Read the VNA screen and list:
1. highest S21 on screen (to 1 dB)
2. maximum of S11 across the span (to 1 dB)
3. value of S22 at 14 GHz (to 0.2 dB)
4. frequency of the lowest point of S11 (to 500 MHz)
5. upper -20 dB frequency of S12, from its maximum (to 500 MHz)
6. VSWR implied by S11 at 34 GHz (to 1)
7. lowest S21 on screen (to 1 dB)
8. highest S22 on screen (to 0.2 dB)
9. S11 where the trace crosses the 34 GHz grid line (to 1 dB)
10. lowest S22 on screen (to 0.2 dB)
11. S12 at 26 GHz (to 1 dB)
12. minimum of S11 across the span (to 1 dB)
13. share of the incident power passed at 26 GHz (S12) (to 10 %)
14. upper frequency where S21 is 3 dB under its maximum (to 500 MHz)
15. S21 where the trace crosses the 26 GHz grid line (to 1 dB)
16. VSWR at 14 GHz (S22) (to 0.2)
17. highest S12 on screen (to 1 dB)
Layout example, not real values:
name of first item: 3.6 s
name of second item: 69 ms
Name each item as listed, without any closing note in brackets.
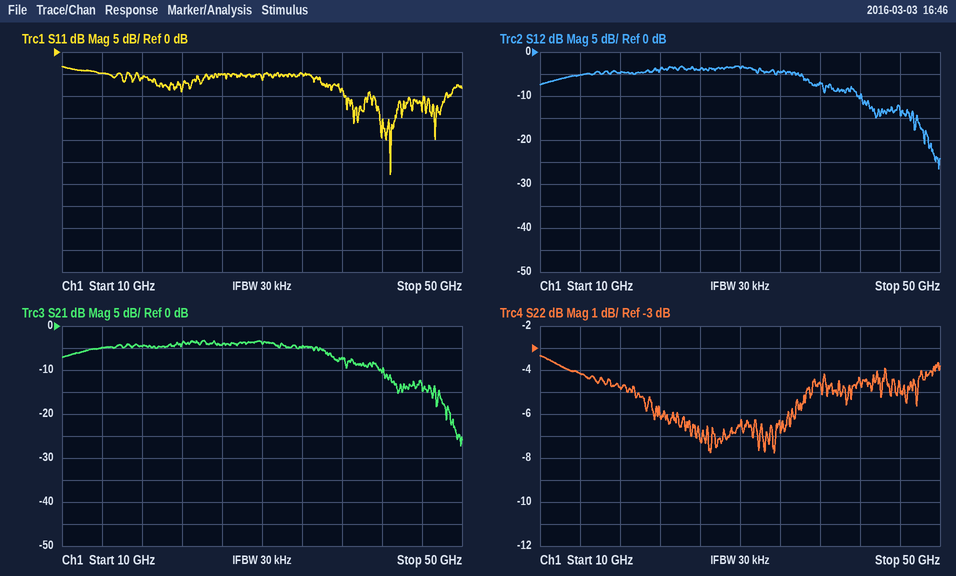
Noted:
highest S21 on screen: -3 dB
maximum of S11 across the span: -3 dB
value of S22 at 14 GHz: -4.2 dB
frequency of the lowest point of S11: 43.0 GHz
upper -20 dB frequency of S12, from its maximum: 49.5 GHz
VSWR implied by S11 at 34 GHz: 4
lowest S21 on screen: -27 dB
highest S22 on screen: -3.4 dB
S11 where the trace crosses the 34 GHz grid line: -5 dB
lowest S22 on screen: -7.8 dB
S12 at 26 GHz: -4 dB
minimum of S11 across the span: -28 dB
share of the incident power passed at 26 GHz (S12): 40 %
upper frequency where S21 is 3 dB under its maximum: 36.5 GHz
S21 where the trace crosses the 26 GHz grid line: -4 dB
VSWR at 14 GHz (S22): 4.2
highest S12 on screen: -3 dB
